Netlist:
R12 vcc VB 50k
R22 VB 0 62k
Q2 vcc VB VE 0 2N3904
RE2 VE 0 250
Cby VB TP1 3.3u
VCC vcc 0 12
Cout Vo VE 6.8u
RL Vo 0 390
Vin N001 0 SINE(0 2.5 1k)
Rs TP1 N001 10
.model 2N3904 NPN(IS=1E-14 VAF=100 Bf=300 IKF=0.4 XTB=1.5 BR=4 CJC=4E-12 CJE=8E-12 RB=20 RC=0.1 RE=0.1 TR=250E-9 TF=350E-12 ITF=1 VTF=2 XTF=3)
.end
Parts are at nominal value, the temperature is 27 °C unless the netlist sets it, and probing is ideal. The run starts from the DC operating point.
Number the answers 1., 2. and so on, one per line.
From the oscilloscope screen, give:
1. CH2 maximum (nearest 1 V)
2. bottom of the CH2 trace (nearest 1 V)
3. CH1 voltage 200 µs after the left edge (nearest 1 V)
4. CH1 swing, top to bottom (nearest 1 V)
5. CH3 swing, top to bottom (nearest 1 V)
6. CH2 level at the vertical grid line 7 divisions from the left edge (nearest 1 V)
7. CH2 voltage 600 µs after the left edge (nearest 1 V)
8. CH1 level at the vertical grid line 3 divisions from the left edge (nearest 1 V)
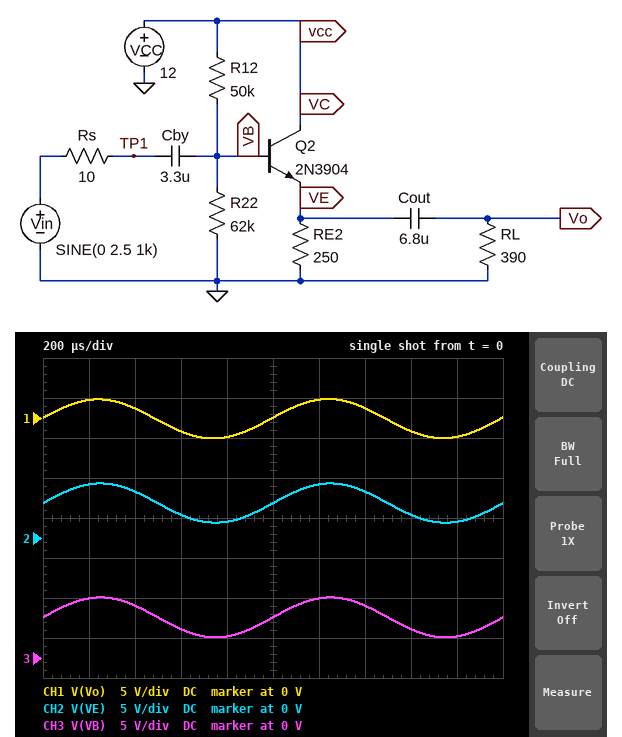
1. 7 V
2. 2 V
3. 2 V
4. 5 V
5. 5 V
6. 6 V
7. 3 V
8. -2 V
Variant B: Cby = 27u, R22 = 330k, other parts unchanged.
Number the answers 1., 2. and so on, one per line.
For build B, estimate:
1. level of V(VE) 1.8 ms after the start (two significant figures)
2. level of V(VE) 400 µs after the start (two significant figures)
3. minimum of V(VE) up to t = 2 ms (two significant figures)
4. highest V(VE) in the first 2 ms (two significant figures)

1. 3.8 V
2. 7.6 V
3. 3.7 V
4. 8.6 V
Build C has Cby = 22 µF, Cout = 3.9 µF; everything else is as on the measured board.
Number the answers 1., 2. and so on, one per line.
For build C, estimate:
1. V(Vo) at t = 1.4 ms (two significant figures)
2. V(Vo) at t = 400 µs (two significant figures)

1. 1.1 V
2. 1.0 V
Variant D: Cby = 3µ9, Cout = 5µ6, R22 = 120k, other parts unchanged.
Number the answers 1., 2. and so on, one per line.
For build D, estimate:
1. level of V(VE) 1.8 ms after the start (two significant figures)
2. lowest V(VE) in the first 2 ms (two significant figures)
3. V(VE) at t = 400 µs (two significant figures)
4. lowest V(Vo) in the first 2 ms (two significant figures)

1. 2.9 V
2. 2.8 V
3. 6.7 V
4. -2.6 V
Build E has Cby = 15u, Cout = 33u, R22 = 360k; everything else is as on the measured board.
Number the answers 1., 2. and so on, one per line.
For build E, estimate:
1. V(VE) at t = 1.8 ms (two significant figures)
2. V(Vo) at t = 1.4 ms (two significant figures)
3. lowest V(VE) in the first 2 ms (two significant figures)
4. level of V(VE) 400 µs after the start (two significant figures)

1. 3.8 V
2. 1.4 V
3. 3.7 V
4. 7.6 V
